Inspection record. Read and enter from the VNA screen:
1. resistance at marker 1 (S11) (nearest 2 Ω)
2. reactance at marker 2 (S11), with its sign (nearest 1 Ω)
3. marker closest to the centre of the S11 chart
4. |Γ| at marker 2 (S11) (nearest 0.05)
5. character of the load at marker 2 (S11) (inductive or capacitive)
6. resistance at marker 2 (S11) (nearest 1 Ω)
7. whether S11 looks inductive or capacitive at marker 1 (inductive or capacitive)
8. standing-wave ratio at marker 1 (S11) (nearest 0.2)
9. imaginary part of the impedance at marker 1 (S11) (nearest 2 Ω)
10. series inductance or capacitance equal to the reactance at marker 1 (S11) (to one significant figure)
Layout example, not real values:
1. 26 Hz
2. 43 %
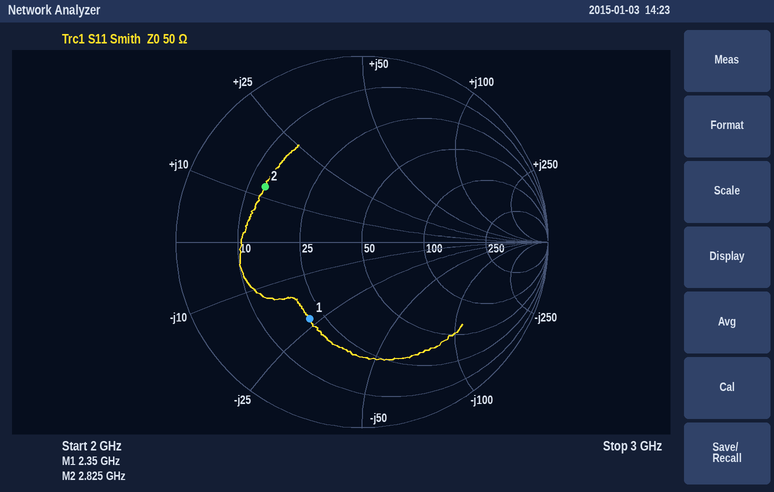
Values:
1. 20 Ω
2. +12 Ω
3. marker 1
4. 0.60
5. inductive
6. 13 Ω
7. capacitive
8. 3.0
9. -22 Ω
10. 3 pF
